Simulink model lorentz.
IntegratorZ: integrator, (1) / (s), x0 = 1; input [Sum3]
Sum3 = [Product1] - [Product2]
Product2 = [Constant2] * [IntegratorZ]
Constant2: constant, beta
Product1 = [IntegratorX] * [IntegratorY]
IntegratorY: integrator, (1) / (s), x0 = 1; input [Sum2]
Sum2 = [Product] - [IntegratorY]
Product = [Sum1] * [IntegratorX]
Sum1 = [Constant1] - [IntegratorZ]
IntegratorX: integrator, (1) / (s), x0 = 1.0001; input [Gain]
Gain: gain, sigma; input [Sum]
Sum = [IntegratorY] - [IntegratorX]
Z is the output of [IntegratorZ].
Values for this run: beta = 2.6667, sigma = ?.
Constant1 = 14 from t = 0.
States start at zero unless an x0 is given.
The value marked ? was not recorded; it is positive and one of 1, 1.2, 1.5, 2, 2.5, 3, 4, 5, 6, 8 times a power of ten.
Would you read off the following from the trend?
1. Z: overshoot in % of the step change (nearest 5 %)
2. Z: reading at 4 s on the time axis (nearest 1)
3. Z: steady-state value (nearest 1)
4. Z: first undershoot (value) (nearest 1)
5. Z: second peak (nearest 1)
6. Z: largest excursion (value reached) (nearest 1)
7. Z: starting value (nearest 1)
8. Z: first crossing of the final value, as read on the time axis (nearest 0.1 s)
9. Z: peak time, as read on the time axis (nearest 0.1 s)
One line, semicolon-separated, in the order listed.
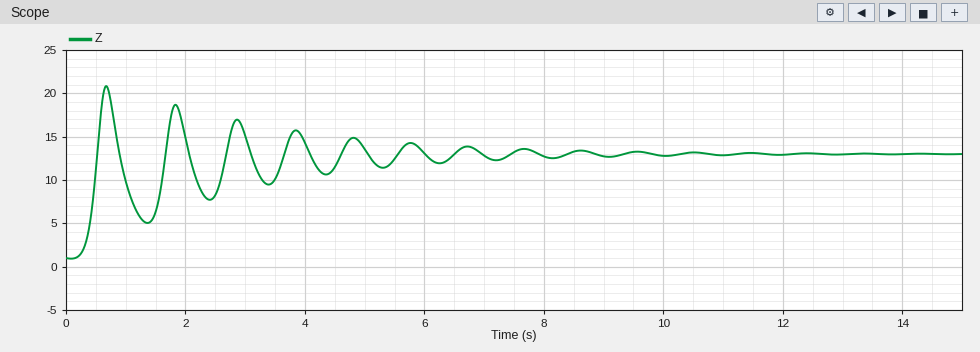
65 %; 14; 13; 5; 19; 21; 1; 0.5 s; 0.7 s
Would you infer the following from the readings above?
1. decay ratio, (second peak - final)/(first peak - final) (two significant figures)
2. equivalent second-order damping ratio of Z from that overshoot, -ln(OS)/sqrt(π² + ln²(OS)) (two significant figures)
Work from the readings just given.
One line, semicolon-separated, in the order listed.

0.75; 0.14
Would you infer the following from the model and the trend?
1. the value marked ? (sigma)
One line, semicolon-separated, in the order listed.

5
